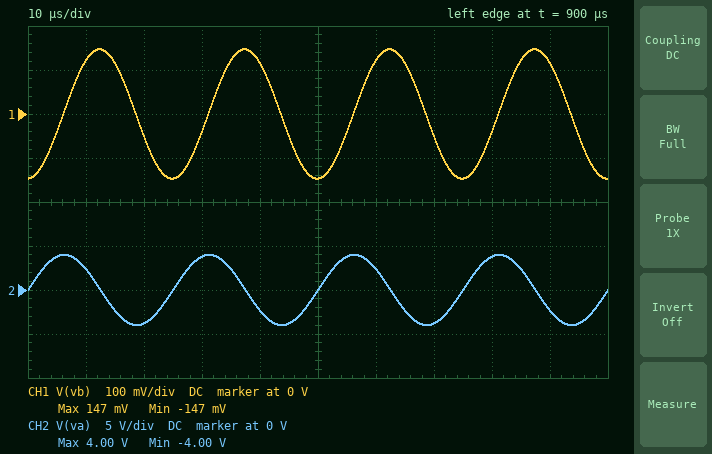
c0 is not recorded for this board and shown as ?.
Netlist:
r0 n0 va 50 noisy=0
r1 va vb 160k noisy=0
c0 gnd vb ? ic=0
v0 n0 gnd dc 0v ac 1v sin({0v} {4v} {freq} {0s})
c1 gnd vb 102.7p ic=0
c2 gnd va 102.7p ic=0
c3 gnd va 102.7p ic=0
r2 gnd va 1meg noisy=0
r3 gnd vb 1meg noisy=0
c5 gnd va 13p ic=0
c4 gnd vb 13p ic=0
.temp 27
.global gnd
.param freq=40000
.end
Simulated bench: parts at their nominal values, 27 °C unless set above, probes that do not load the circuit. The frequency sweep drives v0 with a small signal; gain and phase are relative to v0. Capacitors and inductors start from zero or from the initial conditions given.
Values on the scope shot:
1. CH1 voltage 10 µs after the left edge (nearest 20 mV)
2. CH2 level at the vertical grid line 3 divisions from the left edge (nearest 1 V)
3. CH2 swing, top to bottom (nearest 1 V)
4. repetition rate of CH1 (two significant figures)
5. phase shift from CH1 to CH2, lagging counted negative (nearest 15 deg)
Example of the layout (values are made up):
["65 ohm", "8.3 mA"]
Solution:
["120 mV", "4 V", "8 V", "40 kHz", "90 deg"]
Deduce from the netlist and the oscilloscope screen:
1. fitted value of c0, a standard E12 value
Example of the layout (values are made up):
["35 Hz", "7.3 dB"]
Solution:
["560 pF"]
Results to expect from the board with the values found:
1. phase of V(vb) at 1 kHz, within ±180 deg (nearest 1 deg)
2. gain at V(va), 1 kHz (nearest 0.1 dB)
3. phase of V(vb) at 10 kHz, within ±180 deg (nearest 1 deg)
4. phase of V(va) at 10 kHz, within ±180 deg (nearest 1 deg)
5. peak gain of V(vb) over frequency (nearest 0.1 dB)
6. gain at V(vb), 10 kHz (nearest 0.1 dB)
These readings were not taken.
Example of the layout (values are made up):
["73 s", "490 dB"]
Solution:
["-30 deg", "0 dB", "-80 deg", "0 deg", "-1.3 dB", "-16.8 dB"]
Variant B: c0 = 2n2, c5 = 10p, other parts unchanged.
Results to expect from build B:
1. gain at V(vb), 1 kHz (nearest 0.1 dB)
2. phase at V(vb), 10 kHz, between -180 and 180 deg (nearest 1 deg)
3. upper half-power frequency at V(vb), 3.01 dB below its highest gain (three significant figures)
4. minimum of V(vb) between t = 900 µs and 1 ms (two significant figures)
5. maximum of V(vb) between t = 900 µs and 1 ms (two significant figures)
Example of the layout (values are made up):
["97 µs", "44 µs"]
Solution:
["-8.3 dB", "-87 deg", "498 Hz", "-41 mV", "45 mV"]
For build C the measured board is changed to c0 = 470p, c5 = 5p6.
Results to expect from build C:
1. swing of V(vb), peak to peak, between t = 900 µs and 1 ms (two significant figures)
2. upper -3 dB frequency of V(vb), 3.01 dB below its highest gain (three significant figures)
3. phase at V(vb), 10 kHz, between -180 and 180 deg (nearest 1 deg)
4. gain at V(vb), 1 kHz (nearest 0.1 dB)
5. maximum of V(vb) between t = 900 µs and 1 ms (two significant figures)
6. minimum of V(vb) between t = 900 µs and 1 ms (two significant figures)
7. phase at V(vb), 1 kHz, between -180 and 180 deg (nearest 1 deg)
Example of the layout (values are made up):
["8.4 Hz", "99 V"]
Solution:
["340 mV", "1.97 kHz", "-79 deg", "-2.3 dB", "170 mV", "-170 mV", "-27 deg"]
